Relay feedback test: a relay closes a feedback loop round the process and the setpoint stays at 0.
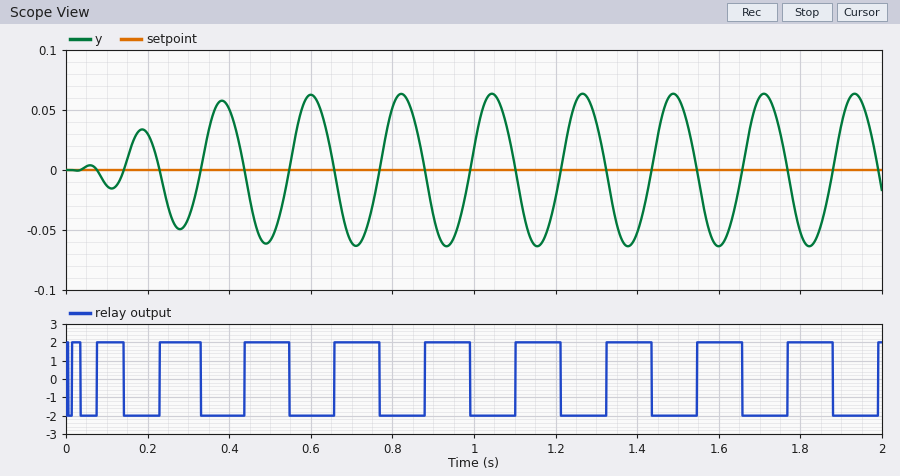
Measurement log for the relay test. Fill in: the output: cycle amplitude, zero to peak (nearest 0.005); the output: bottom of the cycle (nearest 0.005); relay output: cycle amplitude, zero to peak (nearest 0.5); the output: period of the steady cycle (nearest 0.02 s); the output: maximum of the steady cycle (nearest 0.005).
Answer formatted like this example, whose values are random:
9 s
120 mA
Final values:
0.065
-0.065
2.0
0.22 s
0.065
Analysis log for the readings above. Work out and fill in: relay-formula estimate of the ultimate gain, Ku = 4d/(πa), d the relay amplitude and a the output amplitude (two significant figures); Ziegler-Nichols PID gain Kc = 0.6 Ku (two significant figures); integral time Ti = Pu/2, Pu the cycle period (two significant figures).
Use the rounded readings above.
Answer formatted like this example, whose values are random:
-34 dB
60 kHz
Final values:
39
23
0.11 s
